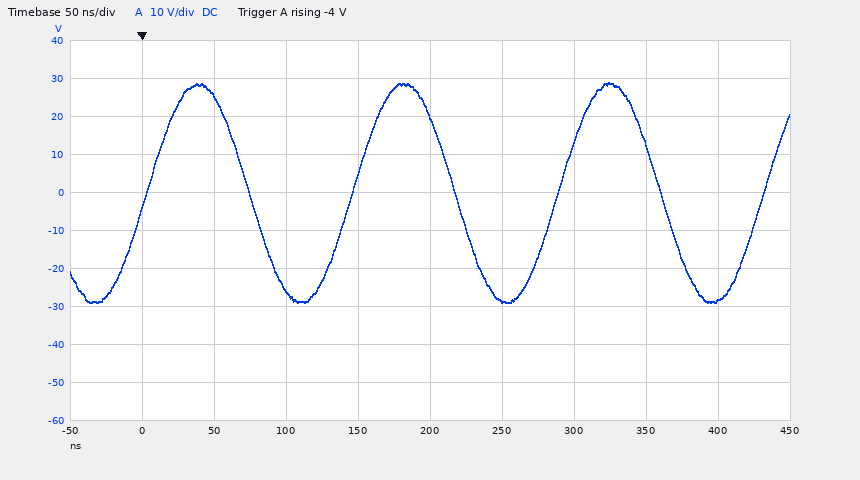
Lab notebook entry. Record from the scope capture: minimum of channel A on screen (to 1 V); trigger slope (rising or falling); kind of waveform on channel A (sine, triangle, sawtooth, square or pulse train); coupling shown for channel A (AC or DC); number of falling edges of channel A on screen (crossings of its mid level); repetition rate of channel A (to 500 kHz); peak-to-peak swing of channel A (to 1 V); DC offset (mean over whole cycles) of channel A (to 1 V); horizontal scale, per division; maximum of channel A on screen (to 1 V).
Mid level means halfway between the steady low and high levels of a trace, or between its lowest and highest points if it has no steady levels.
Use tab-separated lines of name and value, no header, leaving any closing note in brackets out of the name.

minimum of channel A on screen	-29 V
trigger slope	rising
kind of waveform on channel A	sine
coupling shown for channel A	DC
number of falling edges of channel A on screen	3
repetition rate of channel A	7.0 MHz
peak-to-peak swing of channel A	58 V
DC offset (mean over whole cycles) of channel A	0 V
horizontal scale, per division	50 ns
maximum of channel A on screen	29 V
